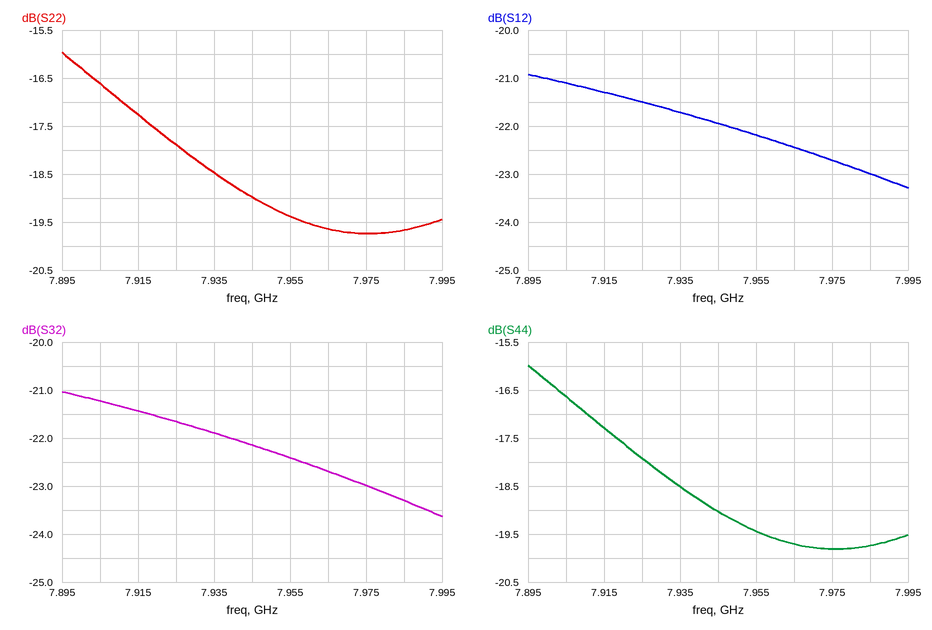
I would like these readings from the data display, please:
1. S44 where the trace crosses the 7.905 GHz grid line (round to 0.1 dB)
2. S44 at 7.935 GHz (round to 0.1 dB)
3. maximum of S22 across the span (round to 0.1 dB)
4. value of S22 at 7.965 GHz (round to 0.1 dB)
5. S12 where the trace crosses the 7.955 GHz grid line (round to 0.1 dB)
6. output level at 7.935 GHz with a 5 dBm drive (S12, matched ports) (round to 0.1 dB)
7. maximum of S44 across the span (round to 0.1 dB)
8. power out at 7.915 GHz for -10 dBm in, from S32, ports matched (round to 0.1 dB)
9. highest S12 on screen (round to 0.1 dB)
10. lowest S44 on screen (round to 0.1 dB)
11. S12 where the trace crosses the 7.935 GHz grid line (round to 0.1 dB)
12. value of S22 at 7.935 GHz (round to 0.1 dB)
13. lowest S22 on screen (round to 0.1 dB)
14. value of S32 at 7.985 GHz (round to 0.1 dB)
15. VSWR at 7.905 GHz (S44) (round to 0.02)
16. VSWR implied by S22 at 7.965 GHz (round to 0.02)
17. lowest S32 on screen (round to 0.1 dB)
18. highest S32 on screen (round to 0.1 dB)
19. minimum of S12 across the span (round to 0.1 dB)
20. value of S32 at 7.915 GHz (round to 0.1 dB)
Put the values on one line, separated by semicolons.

-16.6 dB; -18.5 dB; -16.0 dB; -19.6 dB; -22.2 dB; -16.7 dBm; -16.0 dB; -31.4 dBm; -20.9 dB; -19.8 dB; -21.7 dB; -18.5 dB; -19.7 dB; -23.3 dB; 1.34; 1.24; -23.6 dB; -21.0 dB; -23.3 dB; -21.4 dB
